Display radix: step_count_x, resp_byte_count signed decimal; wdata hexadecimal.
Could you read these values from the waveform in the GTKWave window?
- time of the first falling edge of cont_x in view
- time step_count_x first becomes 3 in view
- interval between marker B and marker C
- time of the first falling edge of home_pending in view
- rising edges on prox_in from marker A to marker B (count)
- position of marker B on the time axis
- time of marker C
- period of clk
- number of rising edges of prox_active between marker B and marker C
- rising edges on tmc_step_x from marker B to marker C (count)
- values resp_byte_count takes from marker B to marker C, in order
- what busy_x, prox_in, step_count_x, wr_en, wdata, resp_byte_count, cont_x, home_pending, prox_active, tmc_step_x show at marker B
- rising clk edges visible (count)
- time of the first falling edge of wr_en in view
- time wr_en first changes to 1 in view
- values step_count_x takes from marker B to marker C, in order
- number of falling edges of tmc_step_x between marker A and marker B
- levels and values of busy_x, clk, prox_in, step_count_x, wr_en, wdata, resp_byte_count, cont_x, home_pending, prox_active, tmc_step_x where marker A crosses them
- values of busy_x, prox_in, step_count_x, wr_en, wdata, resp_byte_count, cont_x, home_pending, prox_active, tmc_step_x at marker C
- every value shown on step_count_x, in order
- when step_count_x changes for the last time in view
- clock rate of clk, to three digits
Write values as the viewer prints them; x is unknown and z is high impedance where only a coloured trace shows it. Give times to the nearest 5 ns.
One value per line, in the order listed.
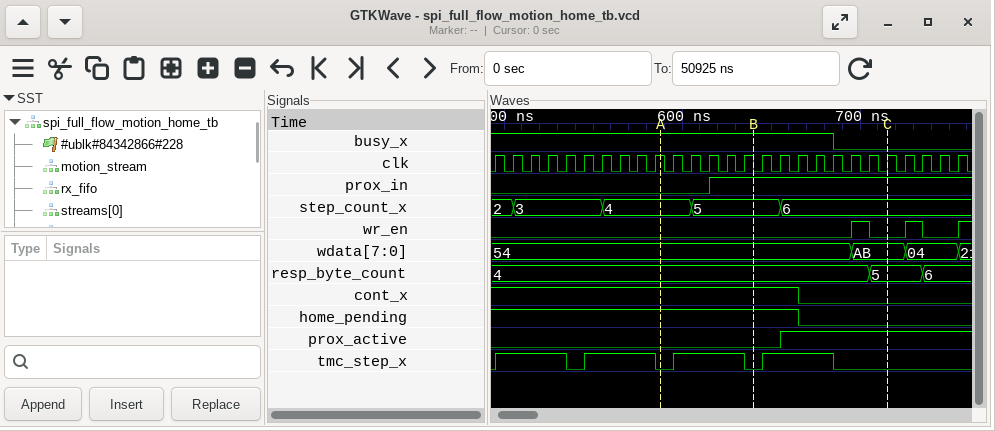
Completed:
665 ns
505 ns
75 ns
665 ns
1
640 ns
715 ns
10 ns
1
1
4, 5
busy_x=1, prox_in=1, step_count_x=5, wr_en=0, wdata=54, resp_byte_count=4, cont_x=1, home_pending=1, prox_active=0, tmc_step_x=0
27
705 ns
695 ns
5, 6
1
busy_x=1, clk=1, prox_in=0, step_count_x=4, wr_en=0, wdata=54, resp_byte_count=4, cont_x=1, home_pending=1, prox_active=0, tmc_step_x=0
busy_x=0, prox_in=1, step_count_x=6, wr_en=0, wdata=AB, resp_byte_count=5, cont_x=0, home_pending=0, prox_active=1, tmc_step_x=0
2, 3, 4, 5, 6
655 ns
100 MHz
